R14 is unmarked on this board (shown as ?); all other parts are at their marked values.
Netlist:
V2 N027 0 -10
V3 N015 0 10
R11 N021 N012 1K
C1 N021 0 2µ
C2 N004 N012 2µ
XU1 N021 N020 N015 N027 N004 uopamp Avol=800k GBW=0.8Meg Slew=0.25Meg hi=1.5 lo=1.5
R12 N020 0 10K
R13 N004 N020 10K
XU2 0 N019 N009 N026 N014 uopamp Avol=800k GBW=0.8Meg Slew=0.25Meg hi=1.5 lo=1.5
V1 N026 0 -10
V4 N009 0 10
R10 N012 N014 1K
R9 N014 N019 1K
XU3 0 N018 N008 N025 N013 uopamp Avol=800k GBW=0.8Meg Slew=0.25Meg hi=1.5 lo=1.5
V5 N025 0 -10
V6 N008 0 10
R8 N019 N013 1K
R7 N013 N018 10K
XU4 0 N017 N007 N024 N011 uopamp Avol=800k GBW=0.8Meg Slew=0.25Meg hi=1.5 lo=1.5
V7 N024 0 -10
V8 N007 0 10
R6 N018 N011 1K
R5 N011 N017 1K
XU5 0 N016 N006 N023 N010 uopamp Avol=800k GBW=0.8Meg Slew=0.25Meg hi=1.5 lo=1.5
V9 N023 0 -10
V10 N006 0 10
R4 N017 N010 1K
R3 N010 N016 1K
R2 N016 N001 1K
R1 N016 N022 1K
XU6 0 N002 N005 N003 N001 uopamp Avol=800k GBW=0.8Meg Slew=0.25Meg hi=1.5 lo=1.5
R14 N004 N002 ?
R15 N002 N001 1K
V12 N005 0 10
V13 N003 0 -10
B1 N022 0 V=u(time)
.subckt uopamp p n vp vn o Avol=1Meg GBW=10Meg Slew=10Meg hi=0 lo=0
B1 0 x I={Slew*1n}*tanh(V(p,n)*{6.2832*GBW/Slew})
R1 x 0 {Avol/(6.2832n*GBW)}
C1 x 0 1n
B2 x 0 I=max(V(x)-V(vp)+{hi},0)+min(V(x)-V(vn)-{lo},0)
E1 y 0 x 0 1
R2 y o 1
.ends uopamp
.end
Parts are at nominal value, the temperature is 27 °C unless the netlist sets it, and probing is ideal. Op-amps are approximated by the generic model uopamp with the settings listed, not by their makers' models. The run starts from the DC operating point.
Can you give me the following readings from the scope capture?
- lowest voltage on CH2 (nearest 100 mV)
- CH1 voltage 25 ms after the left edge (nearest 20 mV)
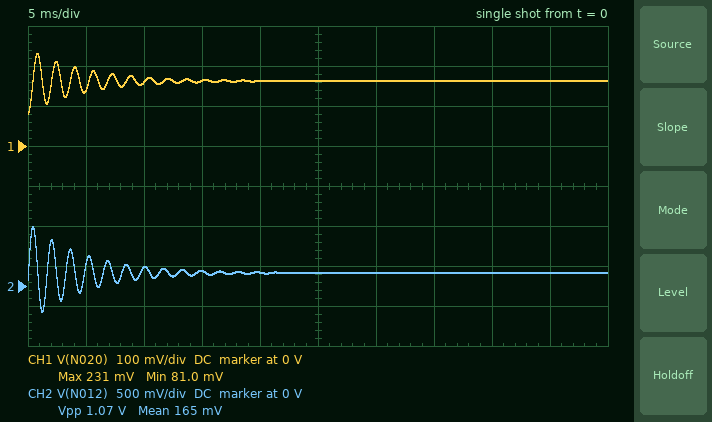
-300 mV
160 mV
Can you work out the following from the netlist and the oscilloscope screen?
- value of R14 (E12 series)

330 Ω
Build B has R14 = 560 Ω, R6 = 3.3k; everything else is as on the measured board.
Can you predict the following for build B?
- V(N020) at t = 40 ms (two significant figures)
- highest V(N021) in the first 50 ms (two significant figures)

260 mV
340 mV
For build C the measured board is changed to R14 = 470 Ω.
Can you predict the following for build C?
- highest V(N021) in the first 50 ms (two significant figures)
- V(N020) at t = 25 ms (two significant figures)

320 mV
230 mV
